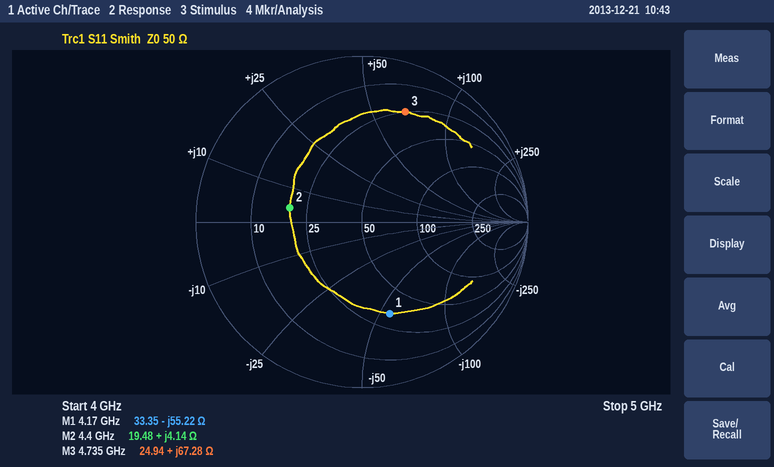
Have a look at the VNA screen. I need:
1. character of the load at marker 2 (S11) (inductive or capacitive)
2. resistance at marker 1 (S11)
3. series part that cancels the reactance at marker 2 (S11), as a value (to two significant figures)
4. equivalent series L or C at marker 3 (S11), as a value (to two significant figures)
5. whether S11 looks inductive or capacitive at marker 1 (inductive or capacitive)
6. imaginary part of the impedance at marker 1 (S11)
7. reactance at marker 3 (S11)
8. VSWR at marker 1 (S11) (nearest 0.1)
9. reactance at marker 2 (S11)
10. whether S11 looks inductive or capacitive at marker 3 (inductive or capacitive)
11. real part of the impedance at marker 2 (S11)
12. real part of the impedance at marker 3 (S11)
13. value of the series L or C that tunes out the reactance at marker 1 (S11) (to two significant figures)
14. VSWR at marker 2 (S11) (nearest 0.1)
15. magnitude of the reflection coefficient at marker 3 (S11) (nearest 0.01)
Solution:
inductive
33.35 Ω
8.7 pF
2.3 nH
capacitive
-55.22 Ω
+67.28 Ω
3.7
+4.14 Ω
inductive
19.48 Ω
24.94 Ω
2.1 nH
2.6
0.71
